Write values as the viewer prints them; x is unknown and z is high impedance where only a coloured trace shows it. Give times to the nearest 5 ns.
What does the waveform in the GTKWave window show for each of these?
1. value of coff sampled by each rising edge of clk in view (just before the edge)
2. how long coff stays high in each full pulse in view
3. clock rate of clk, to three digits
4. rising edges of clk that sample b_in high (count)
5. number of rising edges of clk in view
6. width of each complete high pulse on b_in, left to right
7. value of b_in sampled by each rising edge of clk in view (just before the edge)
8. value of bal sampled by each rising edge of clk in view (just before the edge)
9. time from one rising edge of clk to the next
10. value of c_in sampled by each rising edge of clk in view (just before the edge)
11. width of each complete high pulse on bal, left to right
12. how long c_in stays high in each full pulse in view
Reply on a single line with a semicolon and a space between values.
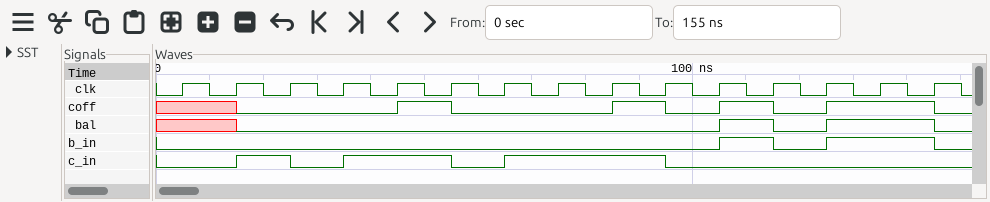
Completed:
x x 0 0 0 1 0 0 0 1 0 1 0 1 1; 10 ns, 10 ns, 10 ns, 20 ns; 100 MHz; 3; 15; 10 ns, 20 ns; 0 0 0 0 0 0 0 0 0 0 0 1 0 1 1; x x 0 0 0 0 0 0 0 0 0 1 0 1 1; 10 ns; 0 0 1 0 1 1 0 1 1 1 0 0 0 0 0; 10 ns, 20 ns; 10 ns, 20 ns, 30 ns
